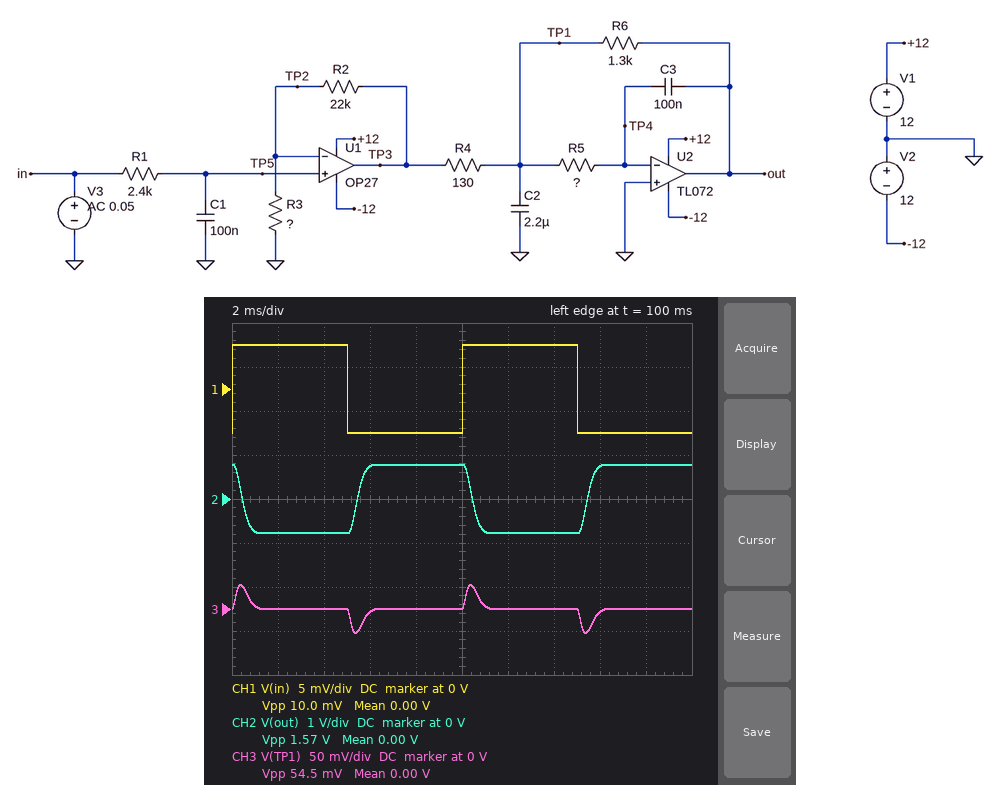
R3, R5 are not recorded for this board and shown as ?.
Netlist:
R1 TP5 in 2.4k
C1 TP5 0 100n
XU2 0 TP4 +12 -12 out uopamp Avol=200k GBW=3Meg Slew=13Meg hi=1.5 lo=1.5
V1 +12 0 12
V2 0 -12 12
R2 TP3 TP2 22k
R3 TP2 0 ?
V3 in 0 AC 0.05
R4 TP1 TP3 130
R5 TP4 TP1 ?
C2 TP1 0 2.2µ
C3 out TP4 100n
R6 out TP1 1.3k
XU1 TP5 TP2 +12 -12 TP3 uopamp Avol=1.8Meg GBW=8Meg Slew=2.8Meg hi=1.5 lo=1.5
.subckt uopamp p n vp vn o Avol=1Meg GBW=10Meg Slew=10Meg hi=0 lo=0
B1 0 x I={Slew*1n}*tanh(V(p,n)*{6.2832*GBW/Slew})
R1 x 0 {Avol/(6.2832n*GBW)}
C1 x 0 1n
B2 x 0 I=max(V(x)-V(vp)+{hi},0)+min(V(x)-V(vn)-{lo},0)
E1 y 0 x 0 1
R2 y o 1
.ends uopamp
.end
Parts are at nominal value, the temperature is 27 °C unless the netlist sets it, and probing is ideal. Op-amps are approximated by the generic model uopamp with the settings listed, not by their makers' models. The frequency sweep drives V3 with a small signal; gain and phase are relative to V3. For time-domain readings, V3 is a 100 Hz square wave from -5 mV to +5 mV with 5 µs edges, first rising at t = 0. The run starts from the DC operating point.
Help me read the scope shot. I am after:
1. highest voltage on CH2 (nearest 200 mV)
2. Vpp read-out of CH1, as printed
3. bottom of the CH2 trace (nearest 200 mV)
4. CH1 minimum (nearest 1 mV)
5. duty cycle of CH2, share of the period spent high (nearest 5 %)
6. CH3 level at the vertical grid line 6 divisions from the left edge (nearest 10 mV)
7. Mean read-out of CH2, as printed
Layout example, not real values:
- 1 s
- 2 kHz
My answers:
- 800 mV
- 10.0 mV
- -800 mV
- -5 mV
- 50 %
- 0 V
- 0.00 V
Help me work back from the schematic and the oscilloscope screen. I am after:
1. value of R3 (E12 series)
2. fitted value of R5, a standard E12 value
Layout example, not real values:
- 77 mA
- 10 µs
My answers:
- 1.5 kΩ
- 100 Ω
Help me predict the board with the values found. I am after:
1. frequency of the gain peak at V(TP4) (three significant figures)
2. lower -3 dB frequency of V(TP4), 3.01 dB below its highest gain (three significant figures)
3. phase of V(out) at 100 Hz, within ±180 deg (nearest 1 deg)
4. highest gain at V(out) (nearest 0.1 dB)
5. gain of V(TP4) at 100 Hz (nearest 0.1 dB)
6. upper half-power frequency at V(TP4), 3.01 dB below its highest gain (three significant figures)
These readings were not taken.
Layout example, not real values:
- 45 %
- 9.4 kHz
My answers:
- 699 Hz
- 335 Hz
- 163 deg
- 43.9 dB
- -45.6 dB
- 1.22 kHz
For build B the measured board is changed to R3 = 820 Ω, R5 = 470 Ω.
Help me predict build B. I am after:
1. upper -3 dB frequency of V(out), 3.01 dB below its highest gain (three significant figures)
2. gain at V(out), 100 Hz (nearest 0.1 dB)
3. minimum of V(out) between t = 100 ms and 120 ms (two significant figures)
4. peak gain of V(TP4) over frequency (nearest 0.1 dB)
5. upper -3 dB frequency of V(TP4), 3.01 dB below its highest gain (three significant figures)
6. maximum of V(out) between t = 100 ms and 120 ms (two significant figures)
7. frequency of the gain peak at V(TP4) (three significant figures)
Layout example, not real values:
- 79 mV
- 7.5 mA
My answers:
- 288 Hz
- 48.5 dB
- -1.4 V
- -34.1 dB
- 690 Hz
- 1.4 V
- 361 Hz
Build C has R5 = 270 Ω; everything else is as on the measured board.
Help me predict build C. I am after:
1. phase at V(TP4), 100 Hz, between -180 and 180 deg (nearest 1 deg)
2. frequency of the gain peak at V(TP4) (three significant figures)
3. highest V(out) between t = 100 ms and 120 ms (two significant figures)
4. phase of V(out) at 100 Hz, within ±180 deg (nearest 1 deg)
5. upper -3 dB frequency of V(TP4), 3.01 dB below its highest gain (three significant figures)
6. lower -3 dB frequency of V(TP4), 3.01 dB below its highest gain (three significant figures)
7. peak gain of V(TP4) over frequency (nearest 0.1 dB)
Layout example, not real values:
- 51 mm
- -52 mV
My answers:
- 57 deg
- 466 Hz
- 800 mV
- 156 deg
- 831 Hz
- 229 Hz
- -36.3 dB
